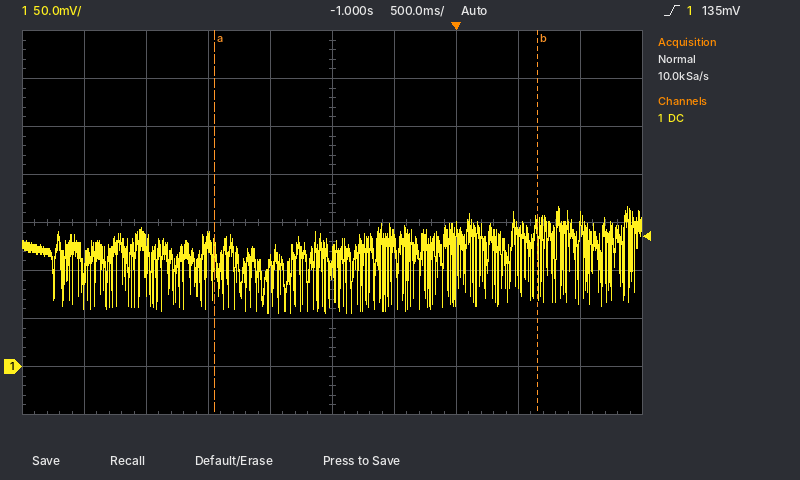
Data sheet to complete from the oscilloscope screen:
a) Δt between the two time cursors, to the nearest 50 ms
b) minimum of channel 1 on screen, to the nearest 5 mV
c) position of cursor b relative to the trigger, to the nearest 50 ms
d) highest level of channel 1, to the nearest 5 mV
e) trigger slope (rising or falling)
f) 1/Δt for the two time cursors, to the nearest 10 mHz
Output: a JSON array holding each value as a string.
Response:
["2.60 s", "55 mV", "+650 ms", "165 mV", "rising", "380 mHz"]
